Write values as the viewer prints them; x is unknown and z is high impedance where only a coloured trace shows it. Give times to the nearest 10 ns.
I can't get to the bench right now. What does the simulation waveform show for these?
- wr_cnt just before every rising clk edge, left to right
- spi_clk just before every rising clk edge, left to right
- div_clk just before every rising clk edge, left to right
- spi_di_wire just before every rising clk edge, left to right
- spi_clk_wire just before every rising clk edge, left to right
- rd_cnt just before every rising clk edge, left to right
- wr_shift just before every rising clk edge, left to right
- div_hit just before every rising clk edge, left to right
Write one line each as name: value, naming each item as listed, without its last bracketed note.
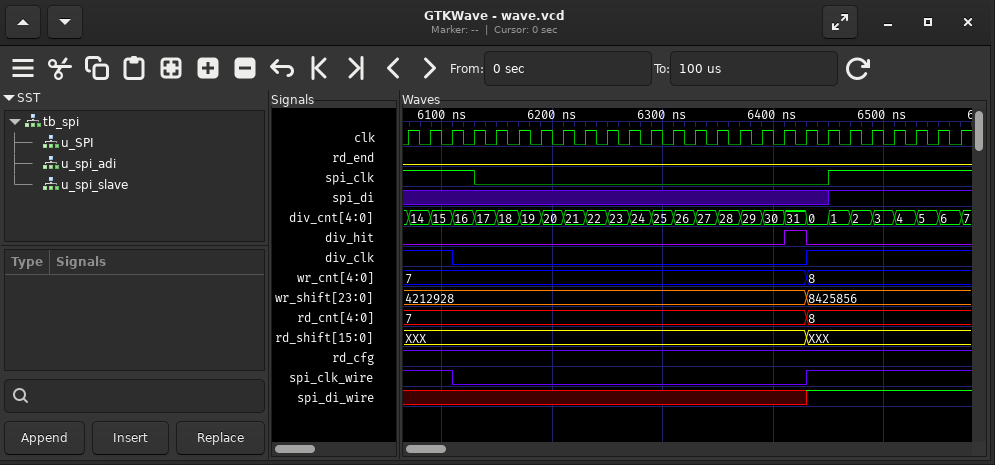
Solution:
wr_cnt just before every rising clk edge, left to right: 7, 7, 7, 7, 7, 7, 7, 7, 7, 7, 7, 7, 7, 7, 7, 7, 7, 7, 7, 8, 8, 8, 8, 8, 8, 8
spi_clk just before every rising clk edge, left to right: 1 1 1 1 0 0 0 0 0 0 0 0 0 0 0 0 0 0 0 0 1 1 1 1 1 1
div_clk just before every rising clk edge, left to right: 1 1 1 0 0 0 0 0 0 0 0 0 0 0 0 0 0 0 0 1 1 1 1 1 1 1
spi_di_wire just before every rising clk edge, left to right: x x x x x x x x x x x x x x x x x x x 1 1 1 1 1 1 1
spi_clk_wire just before every rising clk edge, left to right: 1 1 1 0 0 0 0 0 0 0 0 0 0 0 0 0 0 0 0 1 1 1 1 1 1 1
rd_cnt just before every rising clk edge, left to right: 7, 7, 7, 7, 7, 7, 7, 7, 7, 7, 7, 7, 7, 7, 7, 7, 7, 7, 7, 8, 8, 8, 8, 8, 8, 8
wr_shift just before every rising clk edge, left to right: 4212928, 4212928, 4212928, 4212928, 4212928, 4212928, 4212928, 4212928, 4212928, 4212928, 4212928, 4212928, 4212928, 4212928, 4212928, 4212928, 4212928, 4212928, 4212928, 8425856, 8425856, 8425856, 8425856, 8425856, 8425856, 8425856
div_hit just before every rising clk edge, left to right: 0 0 0 0 0 0 0 0 0 0 0 0 0 0 0 0 0 0 1 0 0 0 0 0 0 0
